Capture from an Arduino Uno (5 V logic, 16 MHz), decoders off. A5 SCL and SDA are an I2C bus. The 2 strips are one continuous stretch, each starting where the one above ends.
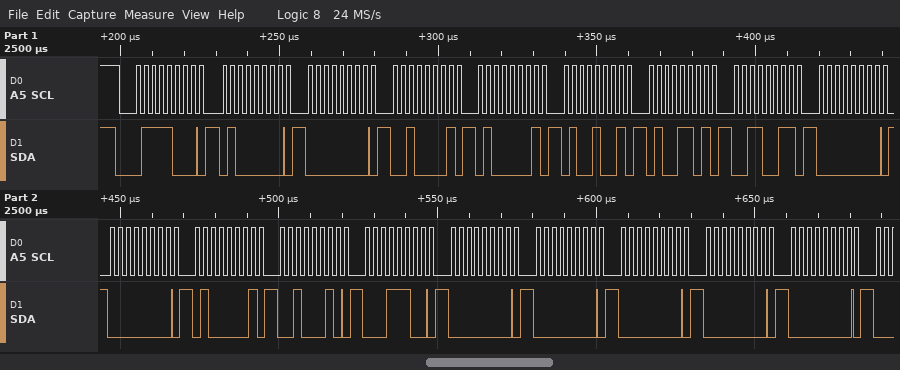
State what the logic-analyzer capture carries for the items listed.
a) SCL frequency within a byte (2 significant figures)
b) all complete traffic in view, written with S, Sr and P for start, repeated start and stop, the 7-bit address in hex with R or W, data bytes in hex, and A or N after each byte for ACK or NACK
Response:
400 kHz
S 3CW A 40 A 00 A 21 A 41 A 49 A 4D A 33 A 00 A 00 A 41 A 22 A 1C A 00 A 00 A 00 A 00 A 00 A
